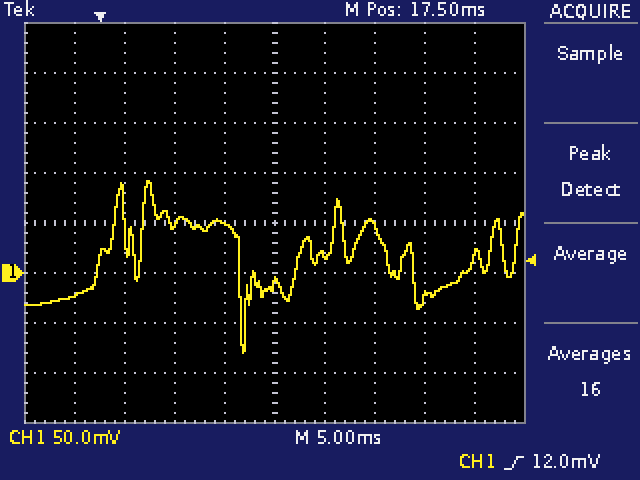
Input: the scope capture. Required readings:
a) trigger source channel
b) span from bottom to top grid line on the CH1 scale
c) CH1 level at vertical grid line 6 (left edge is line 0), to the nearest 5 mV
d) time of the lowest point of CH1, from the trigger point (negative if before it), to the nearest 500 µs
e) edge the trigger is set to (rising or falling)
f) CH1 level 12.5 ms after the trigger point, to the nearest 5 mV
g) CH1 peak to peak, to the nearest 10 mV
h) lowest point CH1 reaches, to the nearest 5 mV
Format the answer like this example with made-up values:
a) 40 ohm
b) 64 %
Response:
a) CH1
b) 400 mV
c) 20 mV
d) +14.5 ms
e) rising
f) 50 mV
g) 170 mV
h) -80 mV
